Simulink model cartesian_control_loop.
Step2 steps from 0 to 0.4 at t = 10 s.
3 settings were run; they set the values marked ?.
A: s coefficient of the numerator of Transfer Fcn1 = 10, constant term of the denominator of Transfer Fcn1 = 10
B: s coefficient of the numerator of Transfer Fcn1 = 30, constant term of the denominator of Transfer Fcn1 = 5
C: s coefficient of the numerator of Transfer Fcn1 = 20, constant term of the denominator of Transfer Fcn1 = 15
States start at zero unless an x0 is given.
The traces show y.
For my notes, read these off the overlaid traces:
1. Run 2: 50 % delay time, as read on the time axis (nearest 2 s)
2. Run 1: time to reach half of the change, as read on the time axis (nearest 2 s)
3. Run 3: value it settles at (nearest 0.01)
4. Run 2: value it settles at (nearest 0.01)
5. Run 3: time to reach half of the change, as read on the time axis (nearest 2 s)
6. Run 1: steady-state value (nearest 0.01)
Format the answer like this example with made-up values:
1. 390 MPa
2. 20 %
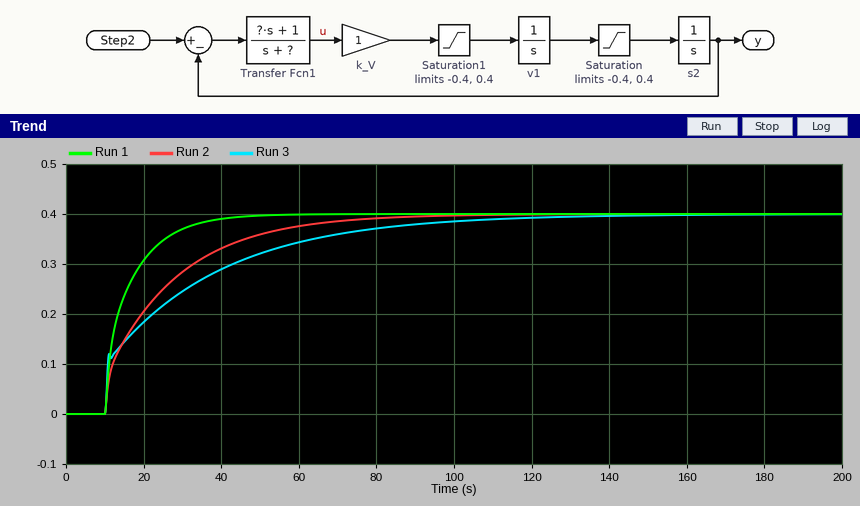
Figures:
1. 20 s
2. 14 s
3. 0.40
4. 0.40
5. 22 s
6. 0.40
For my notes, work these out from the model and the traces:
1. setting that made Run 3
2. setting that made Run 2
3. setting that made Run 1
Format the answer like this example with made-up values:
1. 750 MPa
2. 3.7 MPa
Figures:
1. B
2. C
3. A
